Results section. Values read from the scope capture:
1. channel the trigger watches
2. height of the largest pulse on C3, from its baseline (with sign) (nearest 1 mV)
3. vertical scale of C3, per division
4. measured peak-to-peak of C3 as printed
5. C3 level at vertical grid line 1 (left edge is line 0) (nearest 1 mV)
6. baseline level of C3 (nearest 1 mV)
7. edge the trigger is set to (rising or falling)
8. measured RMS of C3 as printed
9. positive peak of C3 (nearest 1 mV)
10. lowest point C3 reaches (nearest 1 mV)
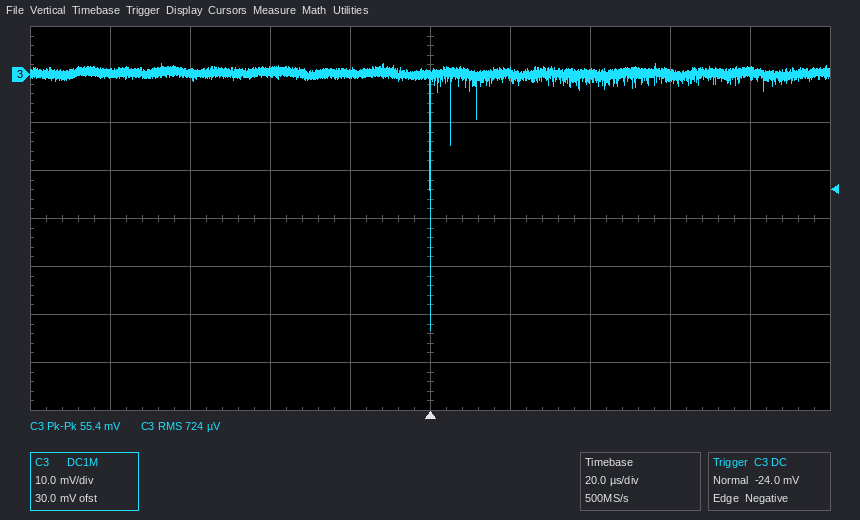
C3
-53 mV
10 mV
55.4 mV
0 mV
0 mV
falling
724 µV
2 mV
-53 mV
